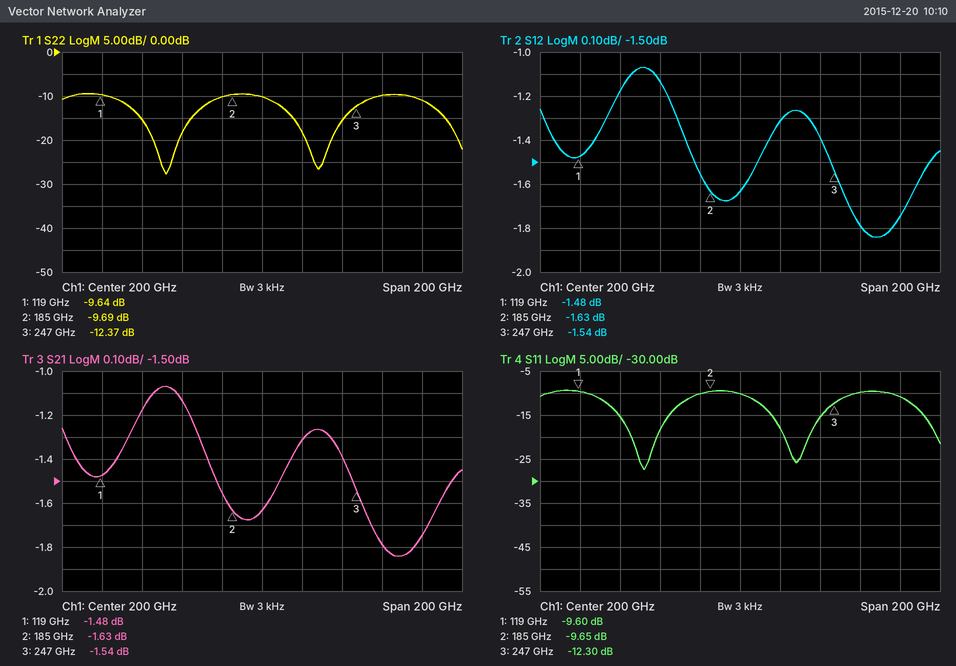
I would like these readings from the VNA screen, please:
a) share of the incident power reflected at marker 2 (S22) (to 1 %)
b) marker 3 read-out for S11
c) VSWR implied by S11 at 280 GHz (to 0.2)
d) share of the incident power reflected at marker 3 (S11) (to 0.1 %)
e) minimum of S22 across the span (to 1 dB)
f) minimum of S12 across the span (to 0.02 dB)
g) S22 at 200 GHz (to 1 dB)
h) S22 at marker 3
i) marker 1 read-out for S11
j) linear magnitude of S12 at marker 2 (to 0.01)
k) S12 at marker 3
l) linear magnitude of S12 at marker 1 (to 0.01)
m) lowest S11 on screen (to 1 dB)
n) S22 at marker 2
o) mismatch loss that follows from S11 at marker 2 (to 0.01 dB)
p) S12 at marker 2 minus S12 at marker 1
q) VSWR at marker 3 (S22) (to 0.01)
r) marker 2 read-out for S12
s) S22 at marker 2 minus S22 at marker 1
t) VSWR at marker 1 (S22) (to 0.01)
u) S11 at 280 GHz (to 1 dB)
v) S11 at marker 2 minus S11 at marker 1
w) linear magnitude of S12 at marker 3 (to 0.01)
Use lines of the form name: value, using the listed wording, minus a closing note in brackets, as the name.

share of the incident power reflected at marker 2 (S22): 11 %
marker 3 read-out for S11: -12.30 dB
VSWR implied by S11 at 280 GHz: 1.8
share of the incident power reflected at marker 3 (S11): 5.9 %
minimum of S22 across the span: -28 dB
minimum of S12 across the span: -1.84 dB
S22 at 200 GHz: -10 dB
S22 at marker 3: -12.37 dB
marker 1 read-out for S11: -9.60 dB
linear magnitude of S12 at marker 2: 0.83
S12 at marker 3: -1.54 dB
linear magnitude of S12 at marker 1: 0.84
lowest S11 on screen: -27 dB
S22 at marker 2: -9.69 dB
mismatch loss that follows from S11 at marker 2: 0.50 dB
S12 at marker 2 minus S12 at marker 1: -0.15 dB
VSWR at marker 3 (S22): 1.63
marker 2 read-out for S12: -1.63 dB
S22 at marker 2 minus S22 at marker 1: -0.05 dB
VSWR at marker 1 (S22): 1.98
S11 at 280 GHz: -11 dB
S11 at marker 2 minus S11 at marker 1: -0.05 dB
linear magnitude of S12 at marker 3: 0.84
